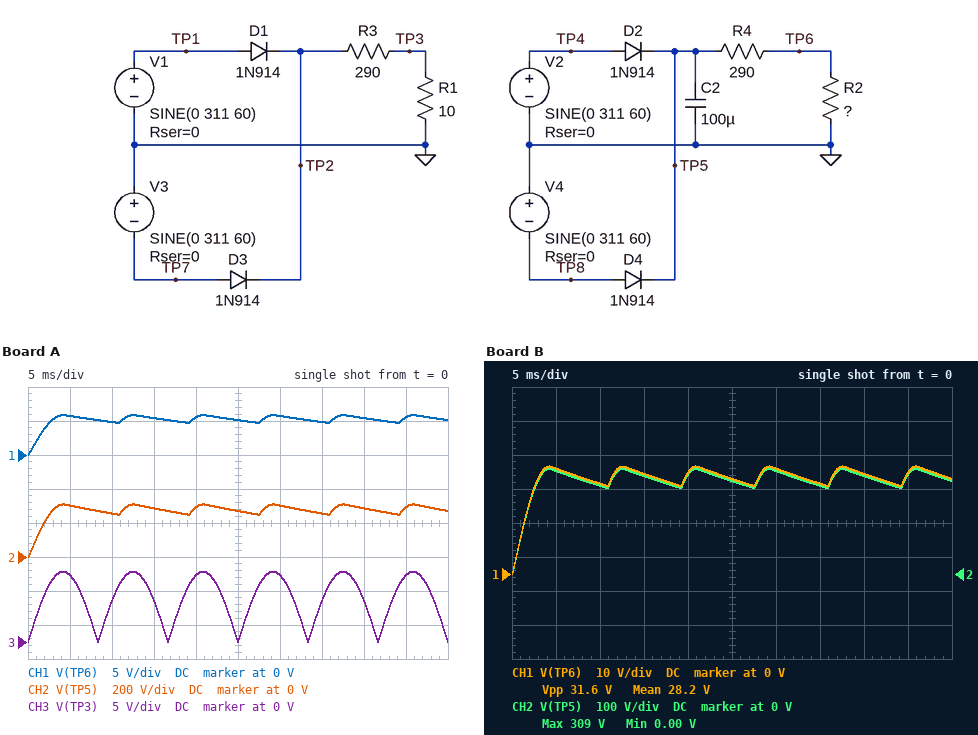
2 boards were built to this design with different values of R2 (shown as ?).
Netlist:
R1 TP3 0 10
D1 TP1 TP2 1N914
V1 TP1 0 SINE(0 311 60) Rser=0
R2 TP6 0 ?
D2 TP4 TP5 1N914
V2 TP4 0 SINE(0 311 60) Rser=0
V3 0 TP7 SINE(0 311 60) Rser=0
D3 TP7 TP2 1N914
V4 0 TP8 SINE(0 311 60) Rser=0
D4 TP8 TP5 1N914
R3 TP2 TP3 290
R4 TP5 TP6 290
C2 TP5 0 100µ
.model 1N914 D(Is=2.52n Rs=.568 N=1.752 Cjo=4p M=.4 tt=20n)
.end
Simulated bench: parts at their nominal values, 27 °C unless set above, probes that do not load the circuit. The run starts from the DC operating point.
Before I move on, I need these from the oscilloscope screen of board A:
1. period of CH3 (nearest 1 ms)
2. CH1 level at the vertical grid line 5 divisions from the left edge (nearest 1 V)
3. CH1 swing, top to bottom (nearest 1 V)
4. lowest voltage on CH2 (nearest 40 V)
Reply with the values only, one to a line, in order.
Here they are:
8 ms
5 V
6 V
0 V
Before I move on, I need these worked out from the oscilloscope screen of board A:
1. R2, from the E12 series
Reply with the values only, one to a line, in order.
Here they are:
5.6 Ω
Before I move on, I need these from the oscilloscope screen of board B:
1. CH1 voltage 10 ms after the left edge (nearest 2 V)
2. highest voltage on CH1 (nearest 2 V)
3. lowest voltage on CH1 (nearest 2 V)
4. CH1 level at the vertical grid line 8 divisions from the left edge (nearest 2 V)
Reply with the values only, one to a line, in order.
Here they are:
26 V
32 V
0 V
30 V
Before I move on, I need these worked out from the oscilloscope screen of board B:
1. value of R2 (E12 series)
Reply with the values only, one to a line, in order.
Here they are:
33 Ω
